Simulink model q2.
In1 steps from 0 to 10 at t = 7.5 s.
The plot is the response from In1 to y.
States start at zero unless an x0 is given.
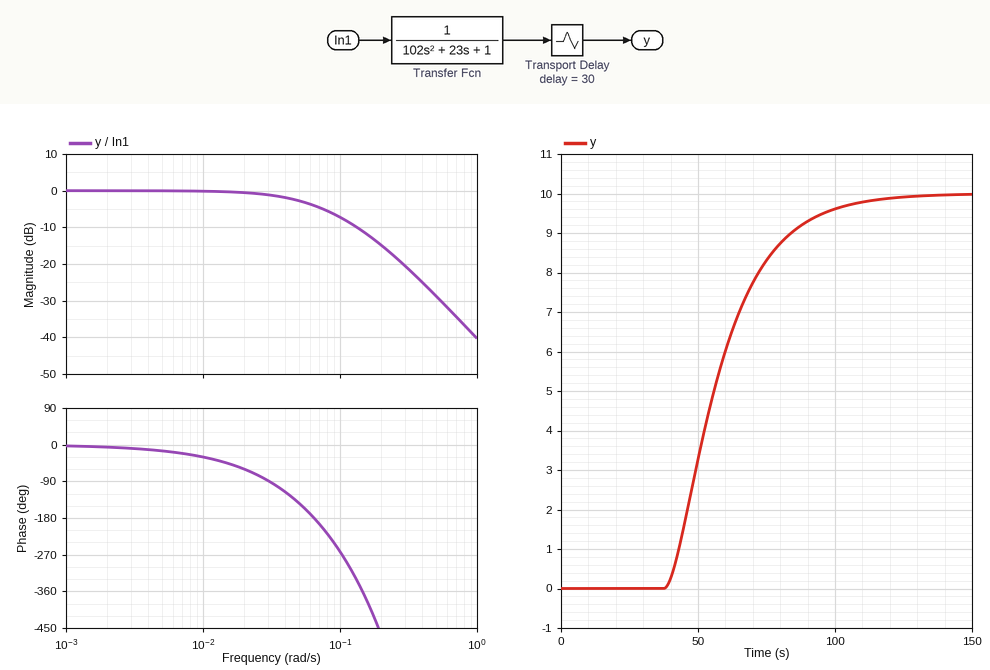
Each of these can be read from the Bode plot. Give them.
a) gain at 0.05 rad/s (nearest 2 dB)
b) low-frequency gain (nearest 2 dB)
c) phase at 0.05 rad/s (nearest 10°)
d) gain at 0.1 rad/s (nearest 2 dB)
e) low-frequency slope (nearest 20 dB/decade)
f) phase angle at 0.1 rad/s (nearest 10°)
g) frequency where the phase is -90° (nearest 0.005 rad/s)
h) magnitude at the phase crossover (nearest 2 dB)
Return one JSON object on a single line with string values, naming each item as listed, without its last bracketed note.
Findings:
{"gain at 0.05 rad/s": "-2 dB", "low-frequency gain": "0 dB", "phase at 0.05 rad/s": "-140°", "gain at 0.1 rad/s": "-8 dB", "low-frequency slope": "0 dB/decade", "phase angle at 0.1 rad/s": "-260°", "frequency where the phase is -90°": "0.030 rad/s", "magnitude at the phase crossover": "-4 dB"}
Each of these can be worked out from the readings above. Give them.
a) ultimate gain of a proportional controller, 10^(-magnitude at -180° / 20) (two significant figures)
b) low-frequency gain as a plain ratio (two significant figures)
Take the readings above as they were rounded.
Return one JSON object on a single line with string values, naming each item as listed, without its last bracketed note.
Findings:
{"ultimate gain of a proportional controller, 10^(-magnitude at -180° / 20)": "1.6", "low-frequency gain as a plain ratio": "1.0"}
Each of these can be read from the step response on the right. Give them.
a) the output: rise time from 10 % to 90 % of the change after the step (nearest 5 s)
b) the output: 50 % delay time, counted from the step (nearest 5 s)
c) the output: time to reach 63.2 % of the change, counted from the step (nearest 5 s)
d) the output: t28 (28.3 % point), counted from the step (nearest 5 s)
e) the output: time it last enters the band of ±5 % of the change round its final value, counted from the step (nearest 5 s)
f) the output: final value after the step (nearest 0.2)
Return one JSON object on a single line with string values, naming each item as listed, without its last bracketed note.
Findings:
{"the output: rise time from 10 % to 90 % of the change after the step": "40 s", "the output: 50 % delay time, counted from the step": "50 s", "the output: time to reach 63.2 % of the change, counted from the step": "55 s", "the output: t28 (28.3 % point), counted from the step": "40 s", "the output: time it last enters the band of ±5 % of the change round its final value, counted from the step": "90 s", "the output: final value after the step": "10.0"}
